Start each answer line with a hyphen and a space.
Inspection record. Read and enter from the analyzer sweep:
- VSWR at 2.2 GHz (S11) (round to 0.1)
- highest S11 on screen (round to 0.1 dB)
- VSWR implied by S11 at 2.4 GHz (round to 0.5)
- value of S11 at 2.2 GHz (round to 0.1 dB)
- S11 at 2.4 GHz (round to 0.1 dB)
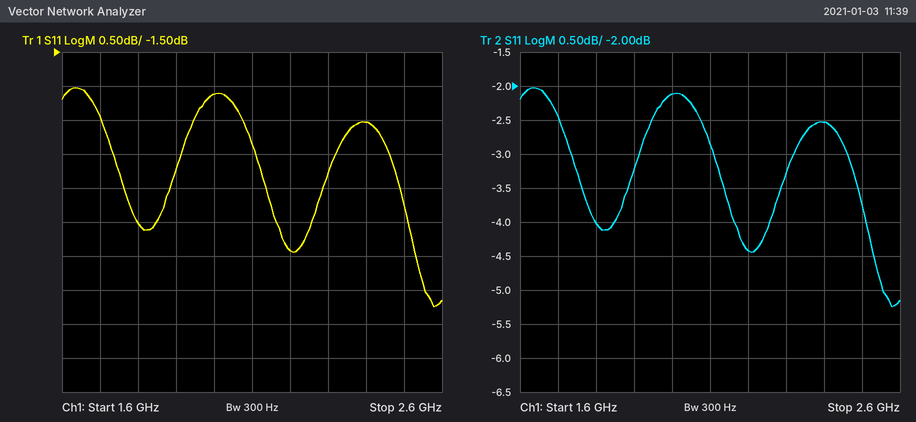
- 4.0
- -2.0 dB
- 7.0
- -4.4 dB
- -2.5 dB
